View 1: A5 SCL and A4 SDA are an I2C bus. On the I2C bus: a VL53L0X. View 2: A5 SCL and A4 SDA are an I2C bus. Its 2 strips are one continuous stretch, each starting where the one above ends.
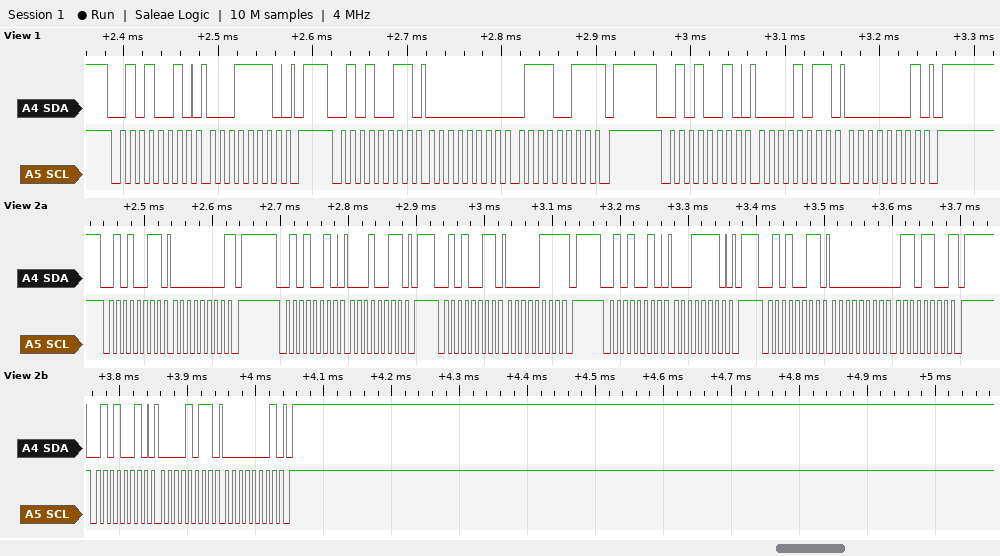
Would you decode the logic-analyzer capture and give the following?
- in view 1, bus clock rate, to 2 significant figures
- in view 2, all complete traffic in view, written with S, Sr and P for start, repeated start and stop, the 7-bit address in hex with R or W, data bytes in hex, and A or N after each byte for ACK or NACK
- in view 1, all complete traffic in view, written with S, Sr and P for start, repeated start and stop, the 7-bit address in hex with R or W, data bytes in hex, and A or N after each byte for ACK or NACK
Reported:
100 kHz
S 29R A 00 N P S 29W A 13 A P S 29R A 07 N P S 29W A 1E A P S 29R A 00 A 6C N P S 29W A 0B A 01 A P
S 29W A 1E A P S 29R A 00 A 73 N P S 29W A 0B A 01 A P
